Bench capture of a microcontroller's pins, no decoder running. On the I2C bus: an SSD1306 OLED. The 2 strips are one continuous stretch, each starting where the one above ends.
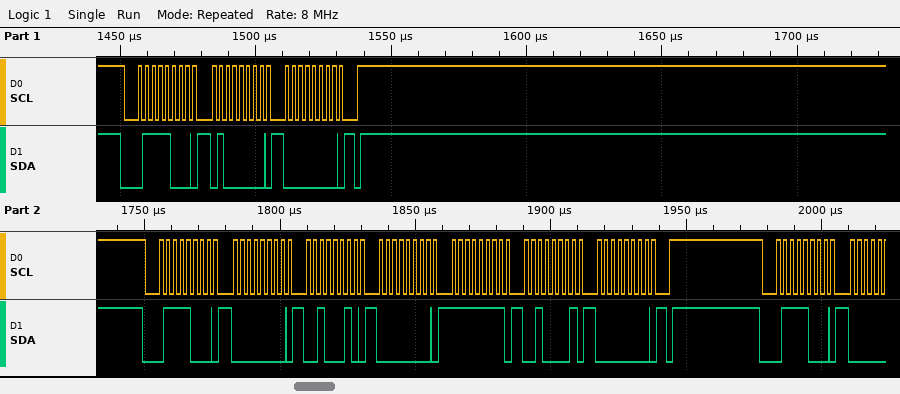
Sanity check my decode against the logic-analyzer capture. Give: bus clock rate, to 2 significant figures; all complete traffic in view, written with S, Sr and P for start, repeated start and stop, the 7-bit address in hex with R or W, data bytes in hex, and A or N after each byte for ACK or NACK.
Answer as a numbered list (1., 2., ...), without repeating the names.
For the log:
1. 400 kHz
2. S 3CW A 40 A 00 A P S 3CW A 00 A 22 A 00 A FF A 21 A 00 A P S 3CW A
